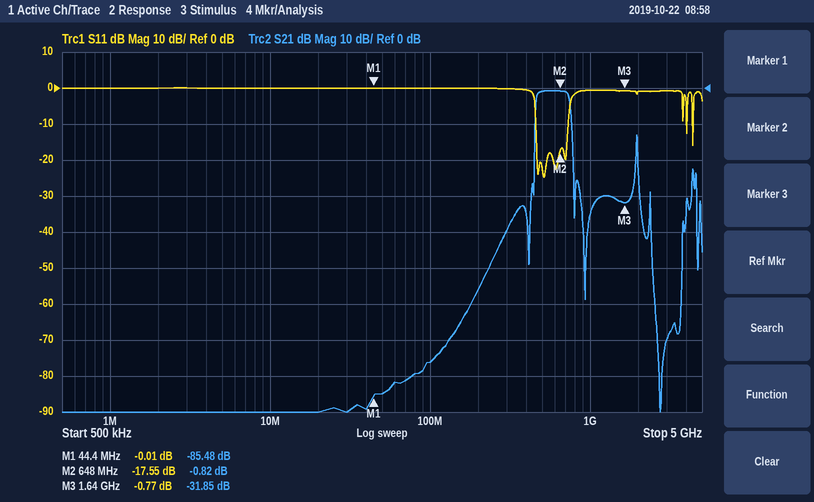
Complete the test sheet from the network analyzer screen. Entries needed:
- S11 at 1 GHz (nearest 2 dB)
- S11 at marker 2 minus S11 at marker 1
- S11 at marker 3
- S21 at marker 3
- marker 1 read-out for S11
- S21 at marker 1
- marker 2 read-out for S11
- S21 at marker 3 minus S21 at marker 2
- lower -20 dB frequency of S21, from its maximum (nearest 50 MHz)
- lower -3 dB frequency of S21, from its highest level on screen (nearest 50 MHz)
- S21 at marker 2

0 dB
-17.54 dB
-0.77 dB
-31.85 dB
-0.01 dB
-85.48 dB
-17.55 dB
-31.03 dB
450 MHz
450 MHz
-0.82 dB
